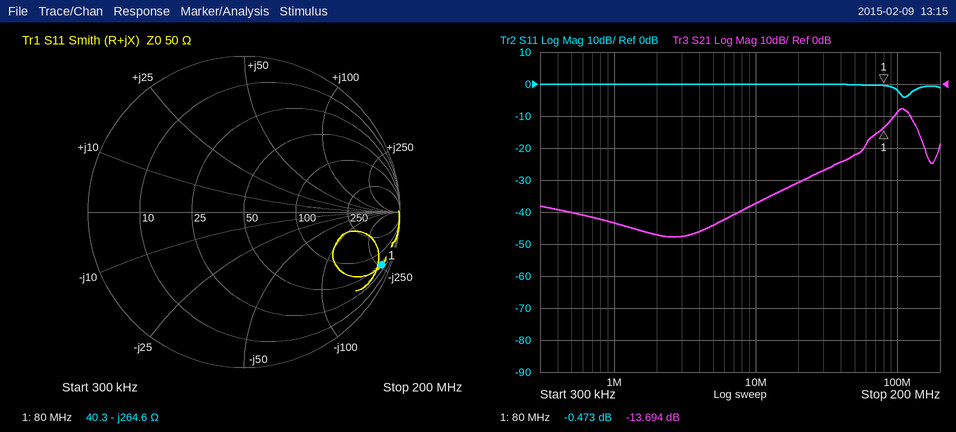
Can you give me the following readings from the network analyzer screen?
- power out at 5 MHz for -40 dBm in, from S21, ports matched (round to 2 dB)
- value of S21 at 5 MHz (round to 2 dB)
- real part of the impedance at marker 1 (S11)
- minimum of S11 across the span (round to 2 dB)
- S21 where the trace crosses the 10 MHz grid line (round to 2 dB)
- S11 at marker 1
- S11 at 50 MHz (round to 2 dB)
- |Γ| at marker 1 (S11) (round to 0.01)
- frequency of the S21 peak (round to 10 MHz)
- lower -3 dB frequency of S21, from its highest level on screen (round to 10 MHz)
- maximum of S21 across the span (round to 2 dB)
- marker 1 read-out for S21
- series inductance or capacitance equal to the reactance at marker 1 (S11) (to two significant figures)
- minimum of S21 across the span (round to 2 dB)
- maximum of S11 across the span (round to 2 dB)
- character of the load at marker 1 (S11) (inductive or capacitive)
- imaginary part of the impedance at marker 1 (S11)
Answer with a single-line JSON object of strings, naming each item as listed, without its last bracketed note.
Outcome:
{"power out at 5 MHz for -40 dBm in, from S21, ports matched": "-84 dBm", "value of S21 at 5 MHz": "-44 dB", "real part of the impedance at marker 1": "40.3 Ω", "minimum of S11 across the span": "-4 dB", "S21 where the trace crosses the 10 MHz grid line": "-38 dB", "S11 at marker 1": "-0.473 dB", "S11 at 50 MHz": "0 dB", "|Γ| at marker 1 (S11)": "0.95", "frequency of the S21 peak": "110 MHz", "lower -3 dB frequency of S21, from its highest level on screen": "90 MHz", "maximum of S21 across the span": "-8 dB", "marker 1 read-out for S21": "-13.694 dB", "series inductance or capacitance equal to the reactance at marker 1 (S11)": "7.5 pF", "minimum of S21 across the span": "-48 dB", "maximum of S11 across the span": "0 dB", "character of the load at marker 1 (S11)": "capacitive", "imaginary part of the impedance at marker 1": "-264.6 Ω"}
